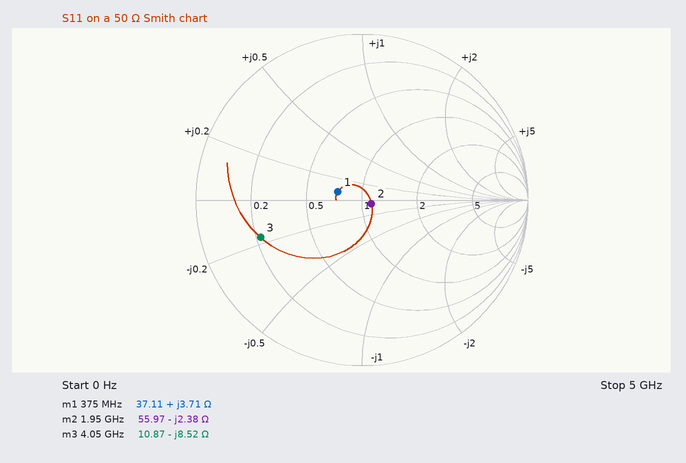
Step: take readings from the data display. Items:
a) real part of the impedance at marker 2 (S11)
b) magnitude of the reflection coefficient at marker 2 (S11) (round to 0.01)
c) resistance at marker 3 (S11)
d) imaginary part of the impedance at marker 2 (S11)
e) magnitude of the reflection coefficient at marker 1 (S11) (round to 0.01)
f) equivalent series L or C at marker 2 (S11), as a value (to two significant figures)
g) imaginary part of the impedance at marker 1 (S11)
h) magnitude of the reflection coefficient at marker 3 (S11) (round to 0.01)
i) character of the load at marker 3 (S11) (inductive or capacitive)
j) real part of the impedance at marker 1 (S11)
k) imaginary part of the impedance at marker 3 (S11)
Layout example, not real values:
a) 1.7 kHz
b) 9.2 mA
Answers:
a) 55.97 Ω
b) 0.06
c) 10.87 Ω
d) -2.38 Ω
e) 0.15
f) 34 pF
g) +3.71 Ω
h) 0.65
i) capacitive
j) 37.11 Ω
k) -8.52 Ω
